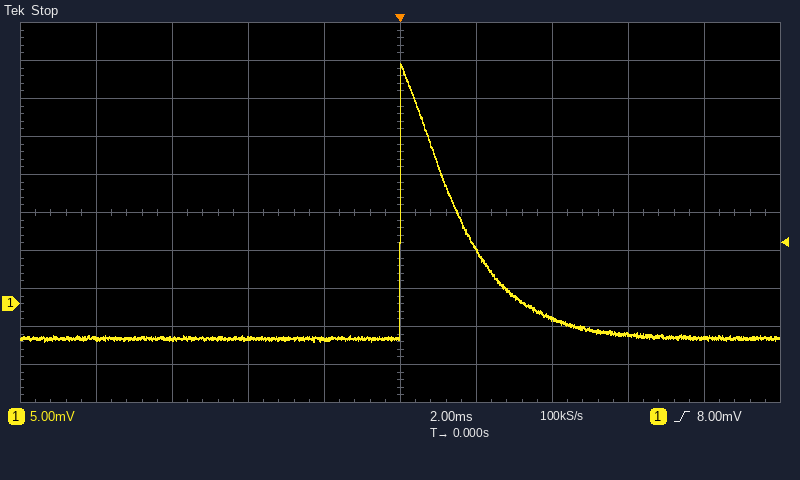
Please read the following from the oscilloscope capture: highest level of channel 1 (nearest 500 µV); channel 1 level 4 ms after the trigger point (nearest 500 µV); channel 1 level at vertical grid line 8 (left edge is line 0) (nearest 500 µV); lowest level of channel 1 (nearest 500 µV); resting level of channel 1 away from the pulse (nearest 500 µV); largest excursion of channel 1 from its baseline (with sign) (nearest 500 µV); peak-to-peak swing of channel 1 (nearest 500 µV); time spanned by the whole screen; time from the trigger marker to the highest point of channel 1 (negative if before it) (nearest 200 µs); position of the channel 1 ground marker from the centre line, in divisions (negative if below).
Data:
31.5 mV
-2.0 mV
-4.0 mV
-5.0 mV
-4.5 mV
+36.0 mV
36.5 mV
20 ms
0.0 ms
-2.4 div
